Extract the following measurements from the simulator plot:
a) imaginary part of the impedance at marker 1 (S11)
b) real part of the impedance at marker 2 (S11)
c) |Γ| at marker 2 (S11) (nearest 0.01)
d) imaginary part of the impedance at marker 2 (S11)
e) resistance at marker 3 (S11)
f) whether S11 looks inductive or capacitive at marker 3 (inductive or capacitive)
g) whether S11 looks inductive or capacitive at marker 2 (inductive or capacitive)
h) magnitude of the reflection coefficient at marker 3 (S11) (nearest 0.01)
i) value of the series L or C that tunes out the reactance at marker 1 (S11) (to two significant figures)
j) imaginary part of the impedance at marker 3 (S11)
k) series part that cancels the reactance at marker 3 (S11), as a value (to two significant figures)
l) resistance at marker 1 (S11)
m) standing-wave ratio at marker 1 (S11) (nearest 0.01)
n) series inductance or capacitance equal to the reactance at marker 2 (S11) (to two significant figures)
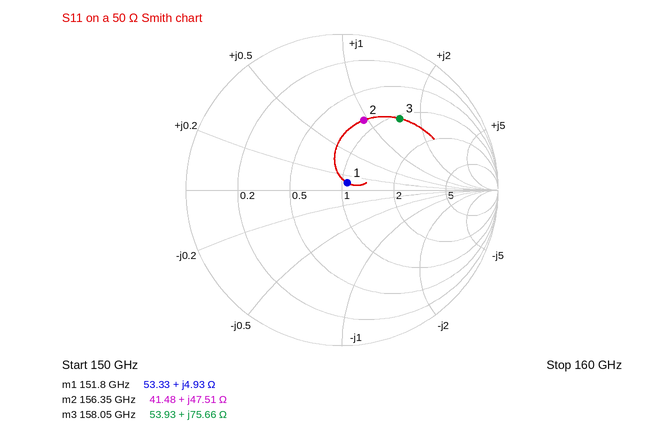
+4.93 Ω
41.48 Ω
0.47
+47.51 Ω
53.93 Ω
inductive
inductive
0.59
210 fF
+75.66 Ω
13 fF
53.33 Ω
1.12
48 pH
